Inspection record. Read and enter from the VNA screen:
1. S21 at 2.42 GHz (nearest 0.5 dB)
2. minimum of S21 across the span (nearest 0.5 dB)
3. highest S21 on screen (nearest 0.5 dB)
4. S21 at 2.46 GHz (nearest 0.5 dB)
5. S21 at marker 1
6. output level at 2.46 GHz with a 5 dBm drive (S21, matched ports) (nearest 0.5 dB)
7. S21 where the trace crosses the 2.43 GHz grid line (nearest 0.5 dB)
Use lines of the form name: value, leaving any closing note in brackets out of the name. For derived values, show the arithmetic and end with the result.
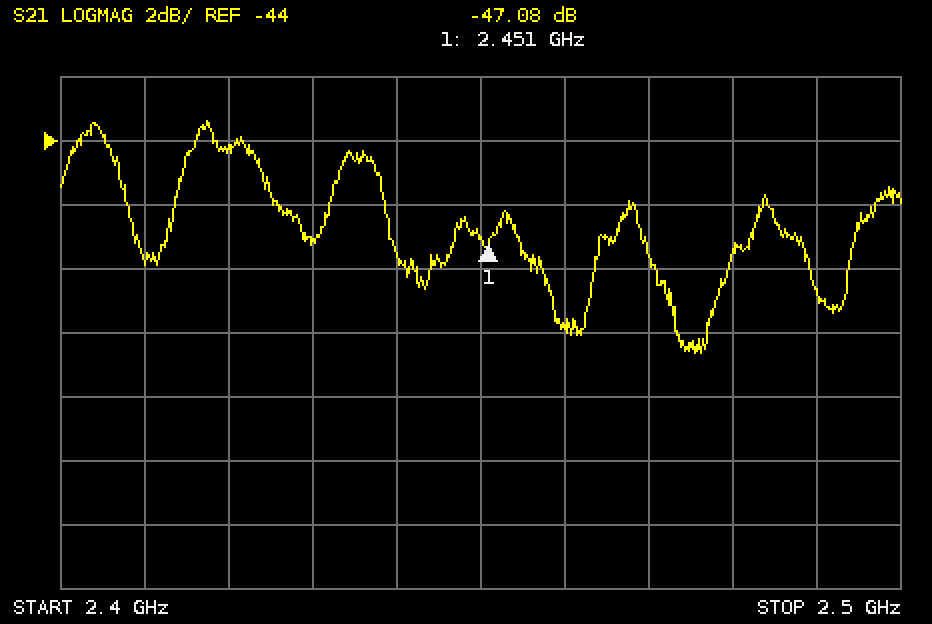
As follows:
S21 at 2.42 GHz: -44.0 dB
minimum of S21 across the span: -50.5 dB
highest S21 on screen: -43.5 dB
S21 at 2.46 GHz: -50.0 dB
S21 at marker 1: -47.08 dB
output level at 2.46 GHz with a 5 dBm drive (S21, matched ports): 5 dBm + (-50.0 dB) = -45.0 dBm
S21 where the trace crosses the 2.43 GHz grid line: -47.0 dB
